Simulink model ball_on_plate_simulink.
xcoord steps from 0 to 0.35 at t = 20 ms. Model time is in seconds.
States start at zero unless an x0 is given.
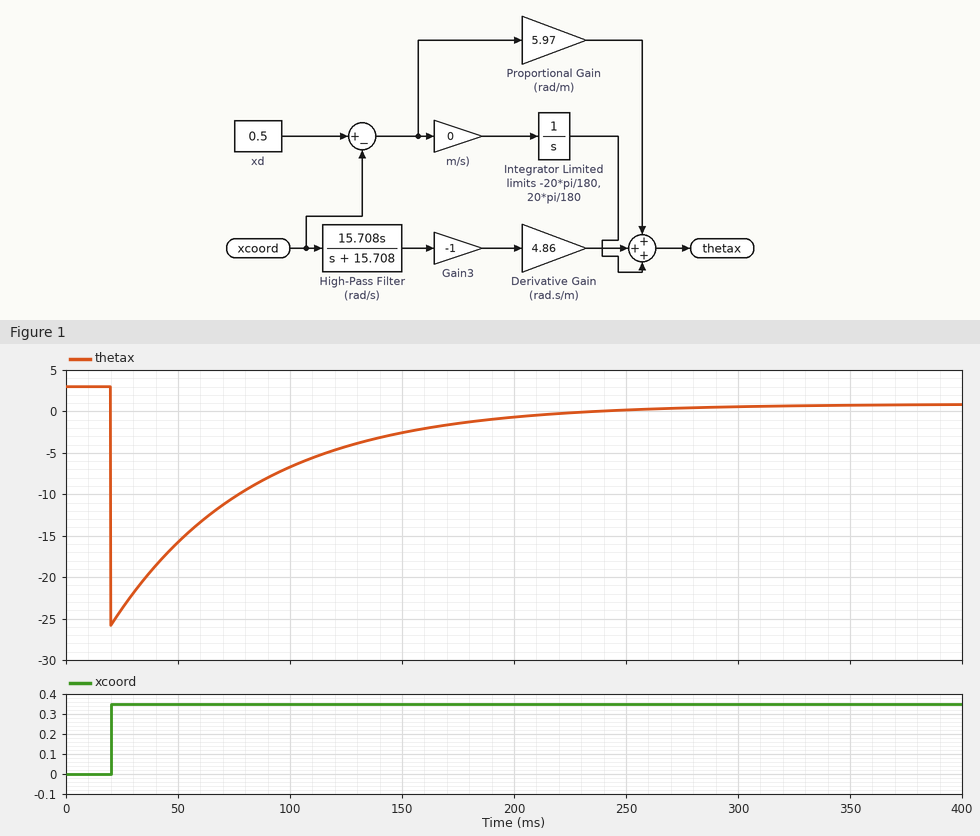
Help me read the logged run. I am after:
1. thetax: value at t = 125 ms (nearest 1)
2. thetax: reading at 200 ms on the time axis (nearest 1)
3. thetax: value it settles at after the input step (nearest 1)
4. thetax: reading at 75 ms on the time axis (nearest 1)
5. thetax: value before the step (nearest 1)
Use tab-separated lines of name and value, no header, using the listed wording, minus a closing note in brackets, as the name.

thetax: value at t = 125 ms	-4
thetax: reading at 200 ms on the time axis	-1
thetax: value it settles at after the input step	1
thetax: reading at 75 ms on the time axis	-10
thetax: value before the step	3
